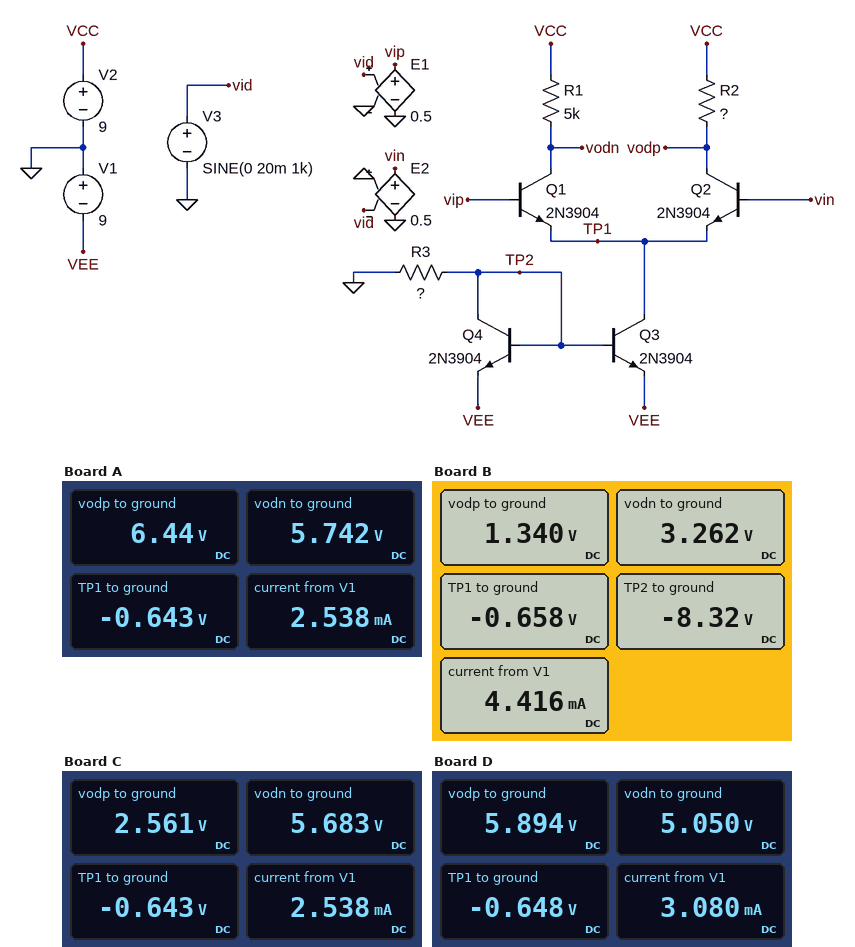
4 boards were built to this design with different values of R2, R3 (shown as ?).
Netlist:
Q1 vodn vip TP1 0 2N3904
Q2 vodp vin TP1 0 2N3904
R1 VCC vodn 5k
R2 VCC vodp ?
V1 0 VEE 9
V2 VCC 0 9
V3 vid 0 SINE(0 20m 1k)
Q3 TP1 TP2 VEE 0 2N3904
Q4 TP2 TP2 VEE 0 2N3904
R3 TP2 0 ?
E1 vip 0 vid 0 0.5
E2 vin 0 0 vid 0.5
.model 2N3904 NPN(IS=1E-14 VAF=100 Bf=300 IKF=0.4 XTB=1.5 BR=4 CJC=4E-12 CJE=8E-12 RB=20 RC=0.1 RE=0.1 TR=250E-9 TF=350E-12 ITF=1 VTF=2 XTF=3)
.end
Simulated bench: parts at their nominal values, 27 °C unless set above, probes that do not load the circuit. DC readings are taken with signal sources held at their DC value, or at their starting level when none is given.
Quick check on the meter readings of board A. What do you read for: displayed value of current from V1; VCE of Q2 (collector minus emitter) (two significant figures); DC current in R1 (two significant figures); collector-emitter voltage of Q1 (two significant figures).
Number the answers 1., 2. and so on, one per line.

1. 2.538 mA
2. 7.1 V
3. 650 µA
4. 6.4 V
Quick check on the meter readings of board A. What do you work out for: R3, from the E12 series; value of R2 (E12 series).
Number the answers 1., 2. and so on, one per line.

1. 6.8 kΩ
2. 3.9 kΩ
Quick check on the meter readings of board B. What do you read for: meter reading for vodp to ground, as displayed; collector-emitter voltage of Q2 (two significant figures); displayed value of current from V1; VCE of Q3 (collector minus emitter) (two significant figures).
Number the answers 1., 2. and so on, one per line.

1. 1.340 V
2. 2.0 V
3. 4.416 mA
4. 8.3 V
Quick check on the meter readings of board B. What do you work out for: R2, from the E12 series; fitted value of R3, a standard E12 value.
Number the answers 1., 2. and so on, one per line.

1. 6.8 kΩ
2. 3.9 kΩ
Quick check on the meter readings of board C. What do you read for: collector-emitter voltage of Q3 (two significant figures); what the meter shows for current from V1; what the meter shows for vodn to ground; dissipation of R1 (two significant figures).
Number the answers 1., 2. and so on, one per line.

1. 8.4 V
2. 2.538 mA
3. 5.683 V
4. 2.2 mW
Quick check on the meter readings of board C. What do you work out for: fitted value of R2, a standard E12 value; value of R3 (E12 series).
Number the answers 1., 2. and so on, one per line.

1. 10 kΩ
2. 6.8 kΩ
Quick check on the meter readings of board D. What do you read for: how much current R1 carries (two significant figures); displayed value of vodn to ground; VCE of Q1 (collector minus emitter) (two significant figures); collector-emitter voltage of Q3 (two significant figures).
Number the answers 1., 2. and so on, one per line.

1. 790 µA
2. 5.050 V
3. 5.7 V
4. 8.4 V
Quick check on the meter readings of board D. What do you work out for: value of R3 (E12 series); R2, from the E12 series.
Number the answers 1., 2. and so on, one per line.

1. 5.6 kΩ
2. 3.9 kΩ
